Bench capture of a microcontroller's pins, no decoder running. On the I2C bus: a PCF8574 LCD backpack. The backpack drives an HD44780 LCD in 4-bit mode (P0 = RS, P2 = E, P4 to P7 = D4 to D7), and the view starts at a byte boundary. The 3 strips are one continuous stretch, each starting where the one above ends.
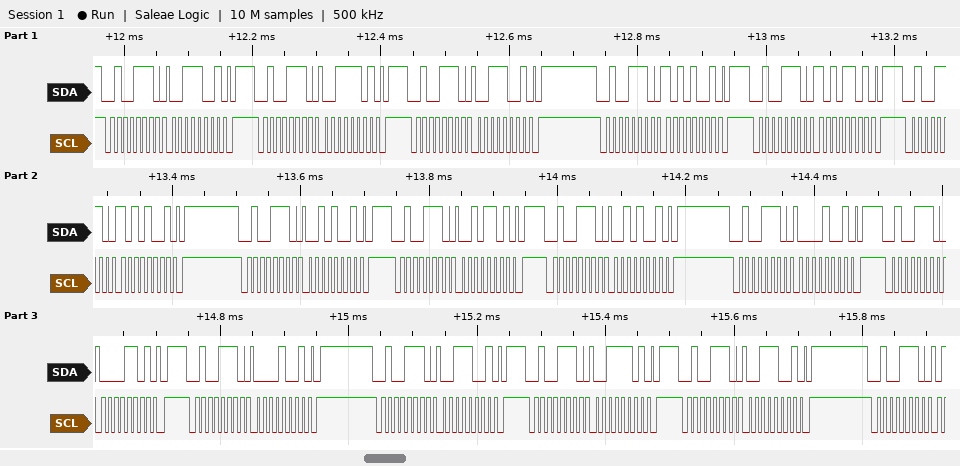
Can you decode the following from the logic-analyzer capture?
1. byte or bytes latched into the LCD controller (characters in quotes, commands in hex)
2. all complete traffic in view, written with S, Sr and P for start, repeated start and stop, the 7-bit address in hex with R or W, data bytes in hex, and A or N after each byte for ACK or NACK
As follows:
':' ' '
S 27W A 39 A P S 27W A 3D A P S 27W A 39 A P S 27W A A9 A P S 27W A AD A P S 27W A A9 A P S 27W A 29 A P S 27W A 2D A P S 27W A 29 A P S 27W A 09 A P S 27W A 0D A P S 27W A 09 A P S 27W A 39 A P S 27W A 3D A P S 27W A 39 A P S 27W A
